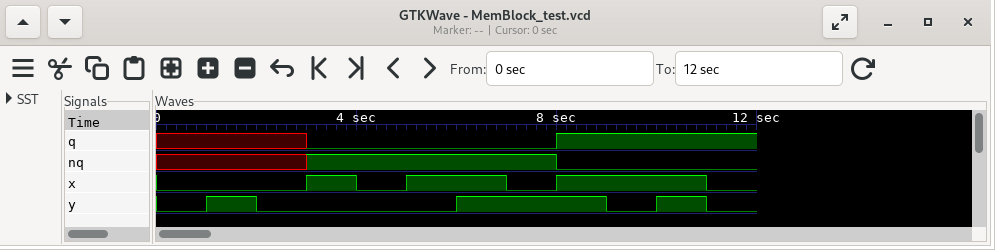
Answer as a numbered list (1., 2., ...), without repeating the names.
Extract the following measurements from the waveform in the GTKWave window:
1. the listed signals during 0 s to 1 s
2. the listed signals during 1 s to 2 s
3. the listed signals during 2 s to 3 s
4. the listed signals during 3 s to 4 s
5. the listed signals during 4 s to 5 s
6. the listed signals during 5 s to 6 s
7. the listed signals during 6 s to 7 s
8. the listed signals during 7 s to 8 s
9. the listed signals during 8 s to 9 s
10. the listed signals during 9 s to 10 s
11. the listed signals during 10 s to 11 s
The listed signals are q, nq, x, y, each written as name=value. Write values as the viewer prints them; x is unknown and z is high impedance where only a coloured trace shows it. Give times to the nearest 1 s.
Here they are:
1. q=x, nq=x, x=0, y=0
2. q=x, nq=x, x=0, y=1
3. q=x, nq=x, x=0, y=0
4. q=0, nq=1, x=1, y=0
5. q=0, nq=1, x=0, y=0
6. q=0, nq=1, x=1, y=0
7. q=0, nq=1, x=1, y=1
8. q=0, nq=1, x=0, y=1
9. q=1, nq=0, x=1, y=1
10. q=1, nq=0, x=1, y=0
11. q=1, nq=0, x=1, y=1
